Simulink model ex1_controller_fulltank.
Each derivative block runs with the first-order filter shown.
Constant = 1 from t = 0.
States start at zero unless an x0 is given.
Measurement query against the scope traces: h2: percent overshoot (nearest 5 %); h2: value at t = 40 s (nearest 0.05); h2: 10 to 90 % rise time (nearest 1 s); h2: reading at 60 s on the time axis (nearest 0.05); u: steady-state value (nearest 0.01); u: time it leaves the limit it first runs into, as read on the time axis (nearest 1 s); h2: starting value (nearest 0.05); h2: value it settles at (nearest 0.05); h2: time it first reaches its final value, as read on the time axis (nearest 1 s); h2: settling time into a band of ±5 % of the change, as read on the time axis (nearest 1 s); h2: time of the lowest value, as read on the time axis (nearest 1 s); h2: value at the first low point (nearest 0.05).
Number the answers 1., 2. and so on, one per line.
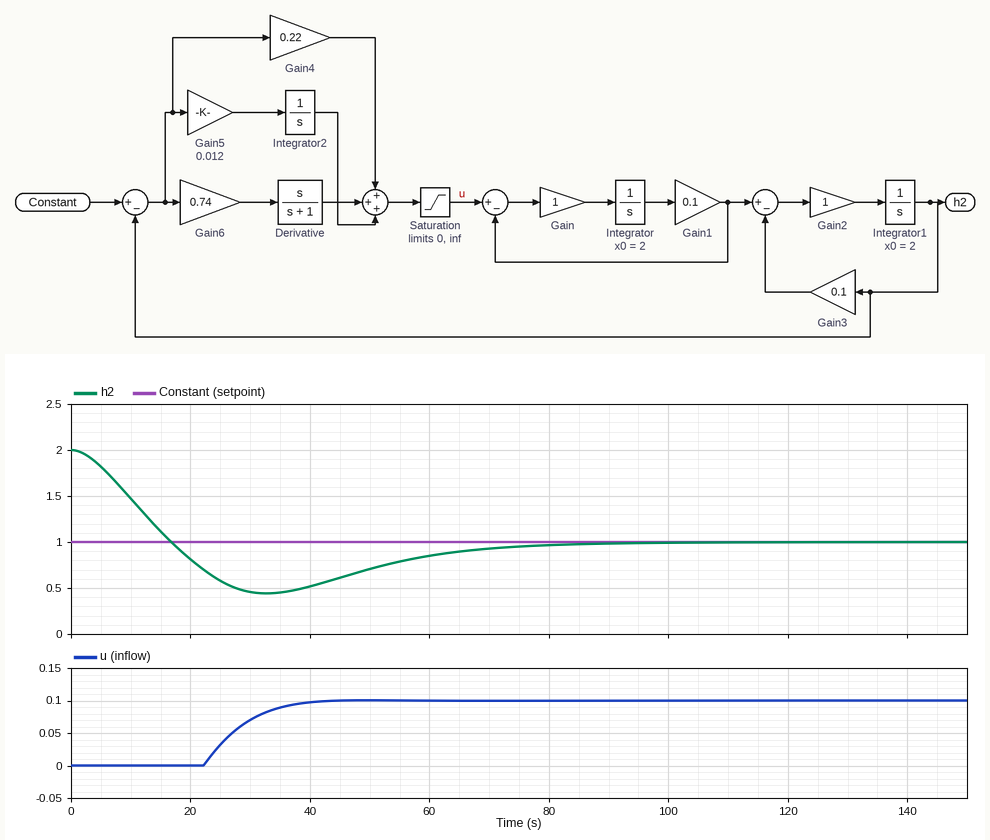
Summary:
1. 55 %
2. 0.50
3. 12 s
4. 0.85
5. 0.10
6. 22 s
7. 2.00
8. 1.00
9. 17 s
10. 75 s
11. 33 s
12. 0.45
